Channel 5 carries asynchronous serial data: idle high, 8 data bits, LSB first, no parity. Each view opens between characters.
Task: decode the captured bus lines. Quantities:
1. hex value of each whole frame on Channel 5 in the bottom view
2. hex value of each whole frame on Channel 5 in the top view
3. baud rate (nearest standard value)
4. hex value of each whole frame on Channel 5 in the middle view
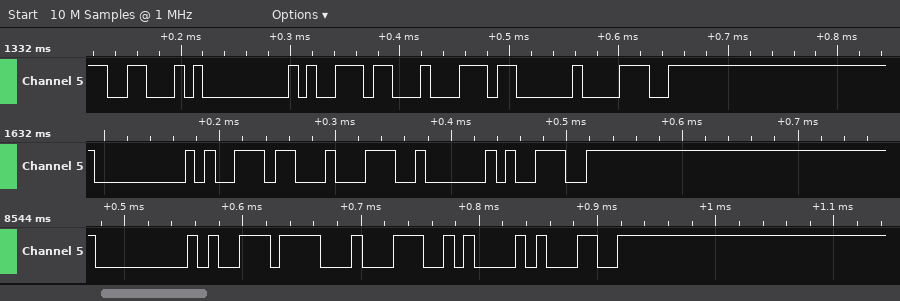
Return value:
00, B9, C4, 0A, 31
46, 00, B9, C4, 03, 38
115200 baud
00, B9, C4, 02, 39
